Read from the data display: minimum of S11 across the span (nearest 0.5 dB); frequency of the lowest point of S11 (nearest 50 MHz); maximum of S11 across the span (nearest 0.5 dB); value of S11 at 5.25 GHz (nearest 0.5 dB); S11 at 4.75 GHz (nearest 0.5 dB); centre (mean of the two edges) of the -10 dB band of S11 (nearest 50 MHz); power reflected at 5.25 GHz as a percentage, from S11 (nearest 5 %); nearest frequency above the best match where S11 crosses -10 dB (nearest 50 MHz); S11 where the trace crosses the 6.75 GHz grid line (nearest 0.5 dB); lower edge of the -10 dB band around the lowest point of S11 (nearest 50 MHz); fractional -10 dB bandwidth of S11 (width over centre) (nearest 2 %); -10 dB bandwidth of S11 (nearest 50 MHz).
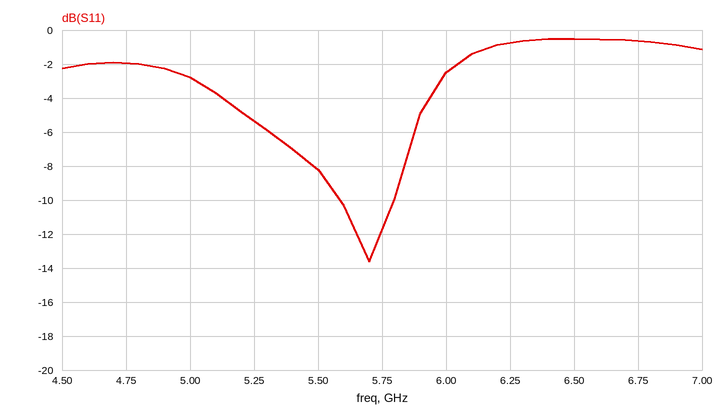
-13.5 dB
5.70 GHz
-0.5 dB
-5.5 dB
-2.0 dB
5.70 GHz
30 %
5.80 GHz
-0.5 dB
5.60 GHz
4 %
200 MHz
